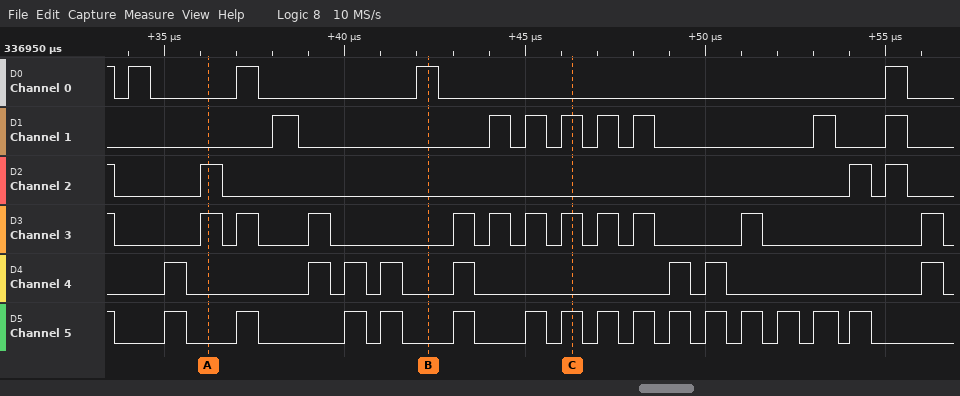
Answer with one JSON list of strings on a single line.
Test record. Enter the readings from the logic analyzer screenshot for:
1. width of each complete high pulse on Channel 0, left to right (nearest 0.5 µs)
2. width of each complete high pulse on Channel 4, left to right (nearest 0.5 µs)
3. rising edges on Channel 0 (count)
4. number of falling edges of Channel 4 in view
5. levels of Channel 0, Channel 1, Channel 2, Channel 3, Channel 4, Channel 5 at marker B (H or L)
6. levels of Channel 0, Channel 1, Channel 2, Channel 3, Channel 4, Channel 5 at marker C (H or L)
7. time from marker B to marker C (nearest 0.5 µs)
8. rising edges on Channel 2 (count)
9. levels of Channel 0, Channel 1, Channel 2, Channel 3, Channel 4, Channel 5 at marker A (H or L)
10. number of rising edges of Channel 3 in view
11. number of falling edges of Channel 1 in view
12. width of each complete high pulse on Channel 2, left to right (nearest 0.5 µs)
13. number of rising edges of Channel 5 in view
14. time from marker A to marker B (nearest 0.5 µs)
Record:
["0.5 µs, 0.5 µs, 0.5 µs, 0.5 µs", "0.5 µs, 0.5 µs, 0.5 µs, 0.5 µs, 0.5 µs, 0.5 µs, 0.5 µs, 0.5 µs", "4", "8", "Channel 0=H, Channel 1=L, Channel 2=L, Channel 3=L, Channel 4=L, Channel 5=L", "Channel 0=L, Channel 1=H, Channel 2=L, Channel 3=H, Channel 4=L, Channel 5=H", "4 µs", "3", "Channel 0=L, Channel 1=L, Channel 2=H, Channel 3=H, Channel 4=L, Channel 5=L", "11", "8", "0.5 µs, 0.5 µs, 0.5 µs", "15", "6 µs"]
